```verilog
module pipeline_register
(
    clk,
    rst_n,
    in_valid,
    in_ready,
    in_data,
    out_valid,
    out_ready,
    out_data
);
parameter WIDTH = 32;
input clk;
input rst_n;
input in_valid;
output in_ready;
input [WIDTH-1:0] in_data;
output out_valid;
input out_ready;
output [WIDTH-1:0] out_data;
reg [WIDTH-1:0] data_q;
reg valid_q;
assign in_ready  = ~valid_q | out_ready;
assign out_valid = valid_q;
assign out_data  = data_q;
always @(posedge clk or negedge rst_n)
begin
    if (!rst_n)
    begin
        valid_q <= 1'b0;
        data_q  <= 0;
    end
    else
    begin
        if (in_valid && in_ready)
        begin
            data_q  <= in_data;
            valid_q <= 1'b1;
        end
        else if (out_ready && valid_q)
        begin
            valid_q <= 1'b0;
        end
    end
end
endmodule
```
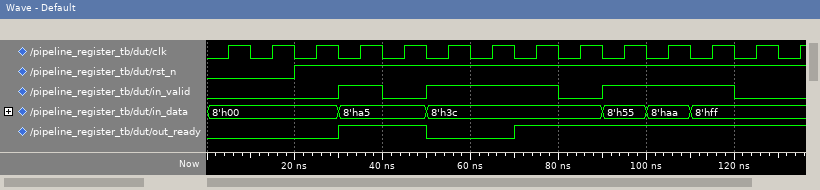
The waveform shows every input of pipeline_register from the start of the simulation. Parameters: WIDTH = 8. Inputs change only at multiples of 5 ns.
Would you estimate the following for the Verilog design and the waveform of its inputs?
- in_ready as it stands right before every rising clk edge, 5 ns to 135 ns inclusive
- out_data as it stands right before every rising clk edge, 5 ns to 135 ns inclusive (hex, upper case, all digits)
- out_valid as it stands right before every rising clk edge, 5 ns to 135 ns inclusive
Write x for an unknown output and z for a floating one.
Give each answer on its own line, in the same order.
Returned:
1 1 1 1 1 1 0 1 1 1 1 1 1 1
00, 00, 00, 00, A5, A5, 3C, 3C, 3C, 3C, 55, AA, FF, FF
0 0 0 0 1 0 1 1 1 0 1 1 1 0
